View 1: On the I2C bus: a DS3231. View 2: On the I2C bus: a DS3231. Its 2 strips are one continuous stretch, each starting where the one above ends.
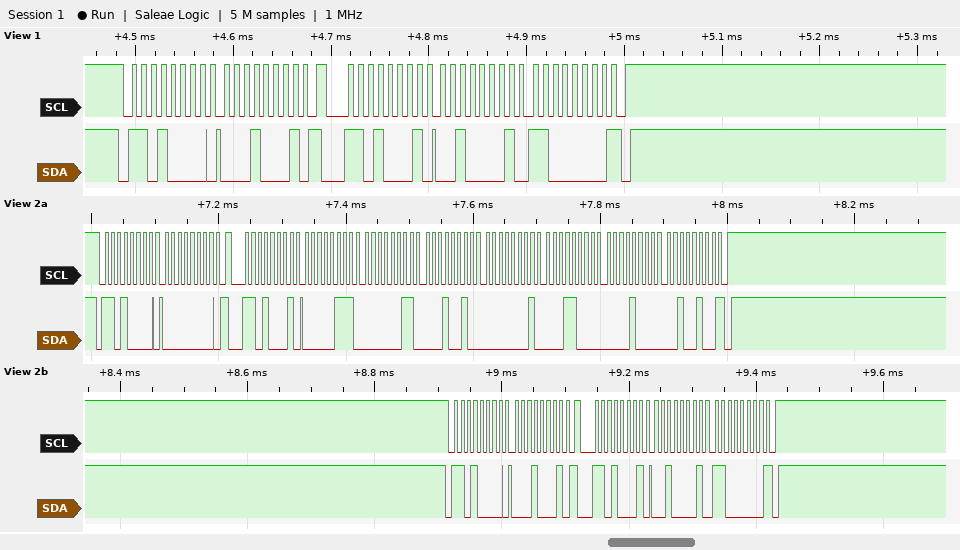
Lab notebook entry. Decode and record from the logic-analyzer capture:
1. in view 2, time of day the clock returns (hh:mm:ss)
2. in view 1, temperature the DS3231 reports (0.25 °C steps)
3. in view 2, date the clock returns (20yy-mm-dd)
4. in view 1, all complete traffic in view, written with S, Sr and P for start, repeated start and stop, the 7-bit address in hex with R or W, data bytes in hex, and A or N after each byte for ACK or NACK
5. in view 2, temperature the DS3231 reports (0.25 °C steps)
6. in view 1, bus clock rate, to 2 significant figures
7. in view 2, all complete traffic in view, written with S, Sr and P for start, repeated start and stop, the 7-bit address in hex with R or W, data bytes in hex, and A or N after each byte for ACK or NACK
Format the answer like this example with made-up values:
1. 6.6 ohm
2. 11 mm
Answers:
1. 12:03:07
2. 33.75 °C
3. 2024-08-18
4. S 68W A 11 A Sr 68R A 21 A C0 N P
5. 33.75 °C
6. 100 kHz
7. S 68W A 00 A Sr 68R A 07 A 03 A 12 A 01 A 18 A 08 A 24 N P S 68W A 11 A Sr 68R A 21 A C0 N P
